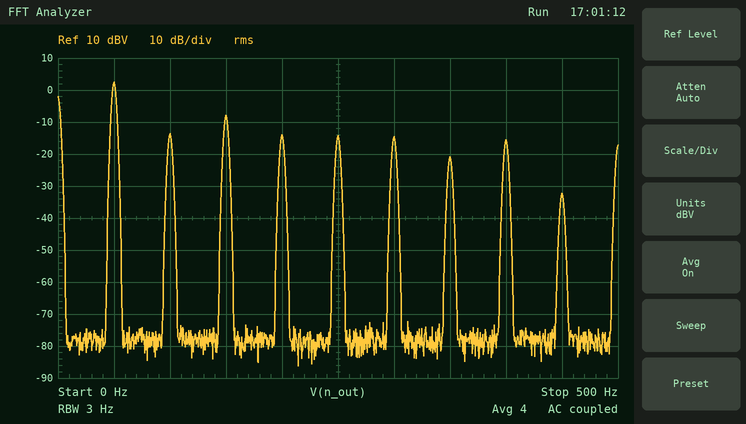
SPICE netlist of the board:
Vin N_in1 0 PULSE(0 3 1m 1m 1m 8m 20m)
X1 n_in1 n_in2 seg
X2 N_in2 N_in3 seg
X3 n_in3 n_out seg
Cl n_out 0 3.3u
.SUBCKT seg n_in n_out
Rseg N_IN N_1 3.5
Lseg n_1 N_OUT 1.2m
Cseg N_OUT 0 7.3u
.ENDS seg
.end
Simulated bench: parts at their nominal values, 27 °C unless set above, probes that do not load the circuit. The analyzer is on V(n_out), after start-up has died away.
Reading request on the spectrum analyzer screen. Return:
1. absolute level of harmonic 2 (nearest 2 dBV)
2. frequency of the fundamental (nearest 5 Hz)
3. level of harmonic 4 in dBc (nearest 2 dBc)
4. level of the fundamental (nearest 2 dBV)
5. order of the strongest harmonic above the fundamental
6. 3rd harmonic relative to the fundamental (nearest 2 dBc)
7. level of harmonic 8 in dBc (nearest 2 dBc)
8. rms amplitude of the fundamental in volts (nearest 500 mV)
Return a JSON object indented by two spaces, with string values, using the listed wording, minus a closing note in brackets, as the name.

{
  "absolute level of harmonic 2": "-14 dBV",
  "frequency of the fundamental": "50 Hz",
  "level of harmonic 4 in dBc": "-16 dBc",
  "level of the fundamental": "2 dBV",
  "order of the strongest harmonic above the fundamental": "3",
  "3rd harmonic relative to the fundamental": "-10 dBc",
  "level of harmonic 8 in dBc": "-18 dBc",
  "rms amplitude of the fundamental in volts": "1.5 V"
}
